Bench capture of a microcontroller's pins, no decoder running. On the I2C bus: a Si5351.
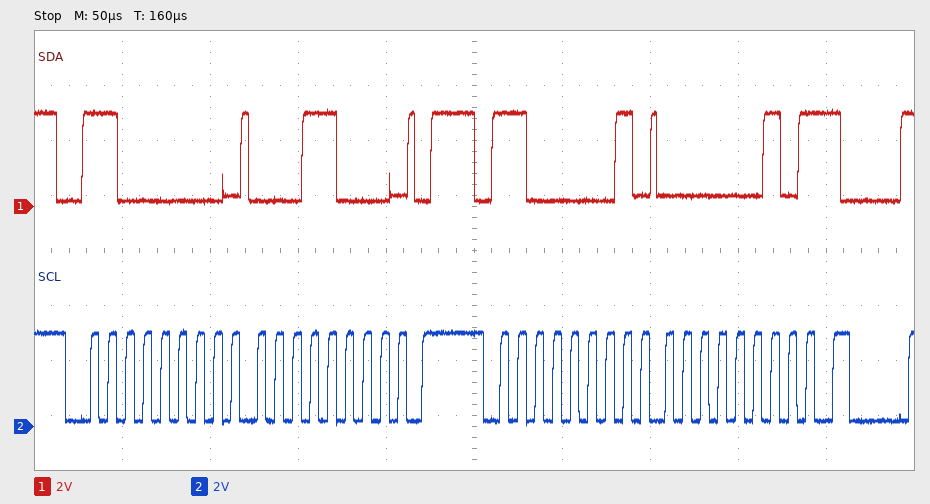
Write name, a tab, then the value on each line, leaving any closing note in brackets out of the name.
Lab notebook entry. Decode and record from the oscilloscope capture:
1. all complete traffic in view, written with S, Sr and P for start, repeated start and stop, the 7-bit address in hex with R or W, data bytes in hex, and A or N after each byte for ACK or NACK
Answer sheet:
all complete traffic in view, written with S, Sr and P for start, repeated start and stop, the 7-bit address in hex with R or W, data bytes in hex, and A or N after each byte for ACK or NACK	S 60W A 18 A P S 60R A 02 N
